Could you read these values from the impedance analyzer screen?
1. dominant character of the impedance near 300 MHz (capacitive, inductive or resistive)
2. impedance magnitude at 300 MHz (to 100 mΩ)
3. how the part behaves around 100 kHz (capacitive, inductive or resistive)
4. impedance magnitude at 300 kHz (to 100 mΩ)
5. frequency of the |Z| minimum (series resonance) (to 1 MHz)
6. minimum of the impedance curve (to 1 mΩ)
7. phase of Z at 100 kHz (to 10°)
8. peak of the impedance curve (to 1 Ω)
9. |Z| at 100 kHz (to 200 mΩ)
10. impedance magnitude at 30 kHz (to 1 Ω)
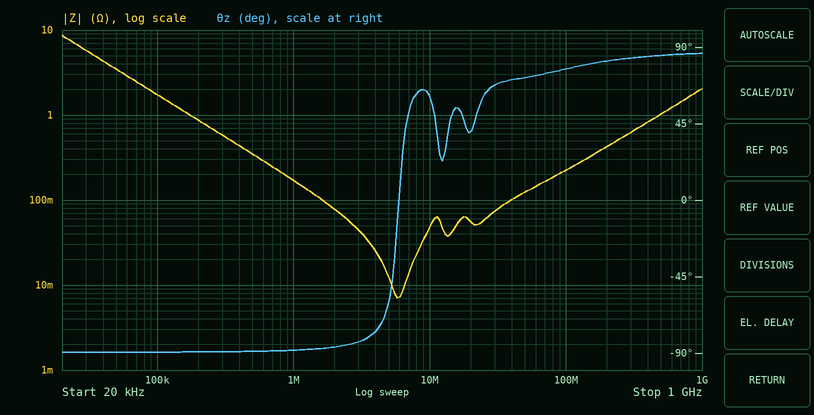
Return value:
inductive
600 mΩ
capacitive
600 mΩ
6 MHz
7 mΩ
-90°
9 Ω
1.8 Ω
6 Ω
